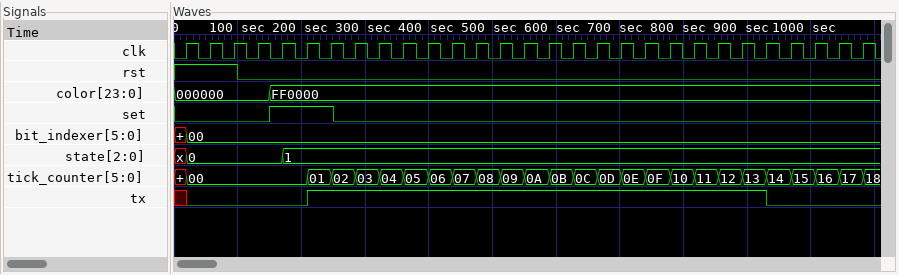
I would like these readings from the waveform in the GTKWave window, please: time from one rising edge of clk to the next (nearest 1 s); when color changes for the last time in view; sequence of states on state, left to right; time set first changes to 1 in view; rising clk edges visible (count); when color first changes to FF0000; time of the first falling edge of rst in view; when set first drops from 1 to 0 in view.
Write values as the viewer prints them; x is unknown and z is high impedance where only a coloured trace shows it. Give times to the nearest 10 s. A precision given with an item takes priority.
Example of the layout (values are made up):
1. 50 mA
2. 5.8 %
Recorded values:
1. 38 s
2. 150 s
3. x, 0, 1
4. 150 s
5. 29
6. 150 s
7. 100 s
8. 250 s
